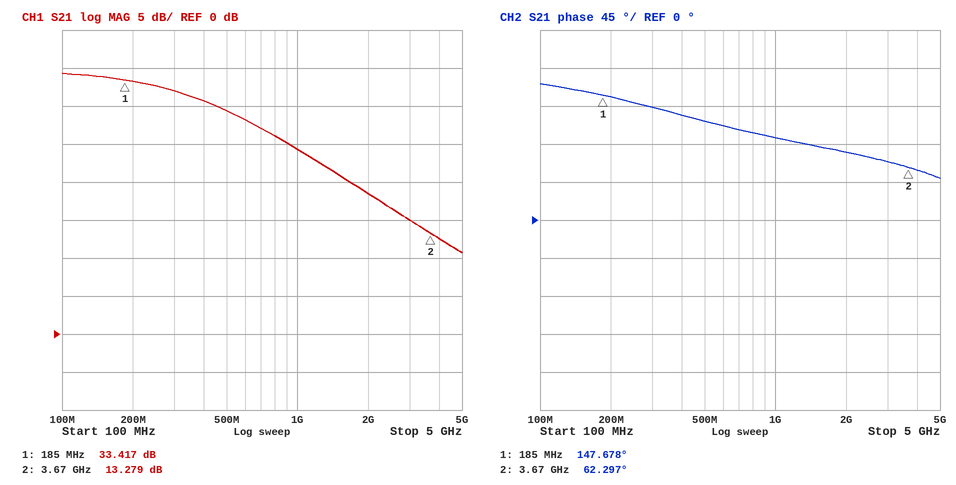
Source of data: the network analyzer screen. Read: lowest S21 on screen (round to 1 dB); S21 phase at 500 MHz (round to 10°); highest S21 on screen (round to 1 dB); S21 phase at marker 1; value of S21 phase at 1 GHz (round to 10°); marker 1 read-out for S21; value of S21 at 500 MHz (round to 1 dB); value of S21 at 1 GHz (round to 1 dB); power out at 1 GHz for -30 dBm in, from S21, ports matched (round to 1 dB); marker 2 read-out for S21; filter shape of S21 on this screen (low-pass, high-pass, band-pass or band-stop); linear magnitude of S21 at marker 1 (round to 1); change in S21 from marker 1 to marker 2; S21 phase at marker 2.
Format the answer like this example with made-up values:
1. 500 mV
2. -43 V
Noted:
1. 11 dB
2. 120°
3. 34 dB
4. 147.678°
5. 100°
6. 33.417 dB
7. 29 dB
8. 24 dB
9. -6 dBm
10. 13.279 dB
11. low-pass
12. 47
13. -20.138 dB
14. 62.297°
